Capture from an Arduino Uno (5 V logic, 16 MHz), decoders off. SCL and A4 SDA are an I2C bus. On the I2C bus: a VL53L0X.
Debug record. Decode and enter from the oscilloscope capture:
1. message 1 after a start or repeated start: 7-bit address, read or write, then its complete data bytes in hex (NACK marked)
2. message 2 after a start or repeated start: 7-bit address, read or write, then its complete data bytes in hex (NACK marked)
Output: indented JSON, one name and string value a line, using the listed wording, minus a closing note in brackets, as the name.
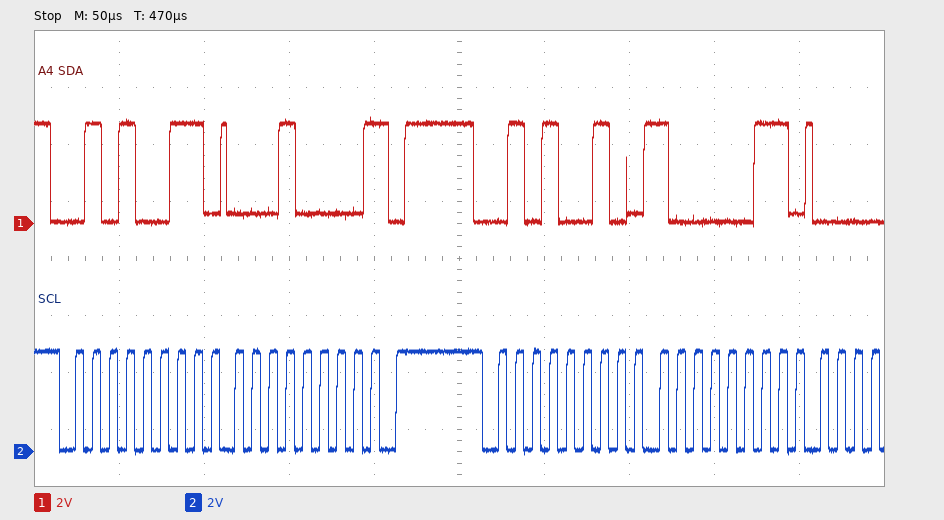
{
  "message 1 after a start or repeated start: 7-bit address, read or write, then its complete data bytes in hex": "0x29 read: 10 NACK",
  "message 2 after a start or repeated start: 7-bit address, read or write, then its complete data bytes in hex": "0x29 write: 83"
}
